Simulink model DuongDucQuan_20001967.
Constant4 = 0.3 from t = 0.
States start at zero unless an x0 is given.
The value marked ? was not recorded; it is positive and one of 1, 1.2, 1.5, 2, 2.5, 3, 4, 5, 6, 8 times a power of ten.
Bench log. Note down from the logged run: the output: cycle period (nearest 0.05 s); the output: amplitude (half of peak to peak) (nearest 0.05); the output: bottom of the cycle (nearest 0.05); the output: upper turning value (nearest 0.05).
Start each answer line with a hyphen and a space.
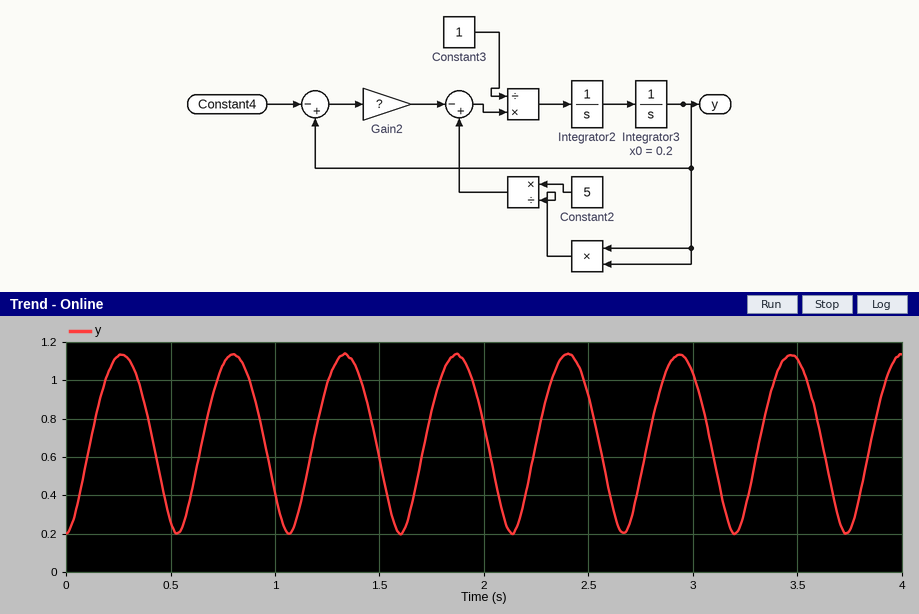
- 0.55 s
- 0.45
- 0.20
- 1.15
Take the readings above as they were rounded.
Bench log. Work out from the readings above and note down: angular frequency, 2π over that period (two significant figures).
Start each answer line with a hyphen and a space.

- 11 rad/s
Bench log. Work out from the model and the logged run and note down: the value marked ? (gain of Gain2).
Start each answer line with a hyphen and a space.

- 60
